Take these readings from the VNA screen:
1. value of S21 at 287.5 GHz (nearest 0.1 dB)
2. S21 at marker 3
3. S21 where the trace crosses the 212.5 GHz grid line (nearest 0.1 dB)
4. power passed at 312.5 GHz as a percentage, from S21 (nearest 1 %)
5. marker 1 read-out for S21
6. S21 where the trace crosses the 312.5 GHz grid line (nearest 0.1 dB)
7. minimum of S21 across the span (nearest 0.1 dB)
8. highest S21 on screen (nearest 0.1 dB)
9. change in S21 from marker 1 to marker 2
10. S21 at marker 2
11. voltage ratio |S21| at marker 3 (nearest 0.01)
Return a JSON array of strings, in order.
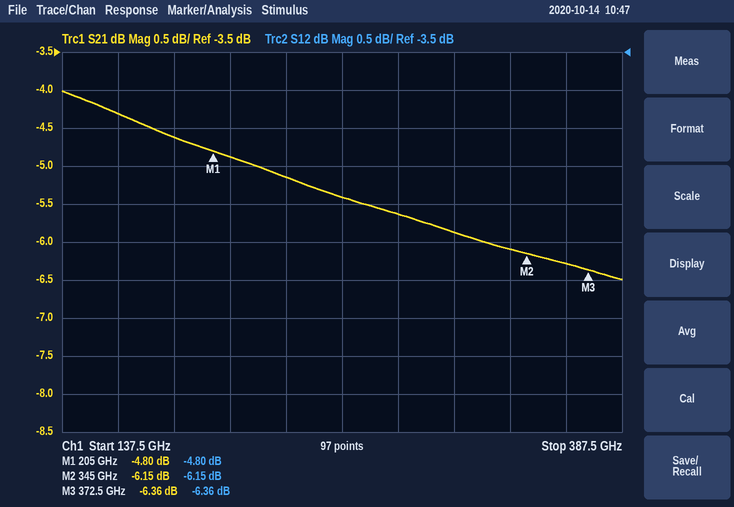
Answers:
["-5.6 dB", "-6.36 dB", "-4.9 dB", "26 %", "-4.80 dB", "-5.9 dB", "-6.5 dB", "-4.0 dB", "-1.35 dB", "-6.15 dB", "0.48"]
